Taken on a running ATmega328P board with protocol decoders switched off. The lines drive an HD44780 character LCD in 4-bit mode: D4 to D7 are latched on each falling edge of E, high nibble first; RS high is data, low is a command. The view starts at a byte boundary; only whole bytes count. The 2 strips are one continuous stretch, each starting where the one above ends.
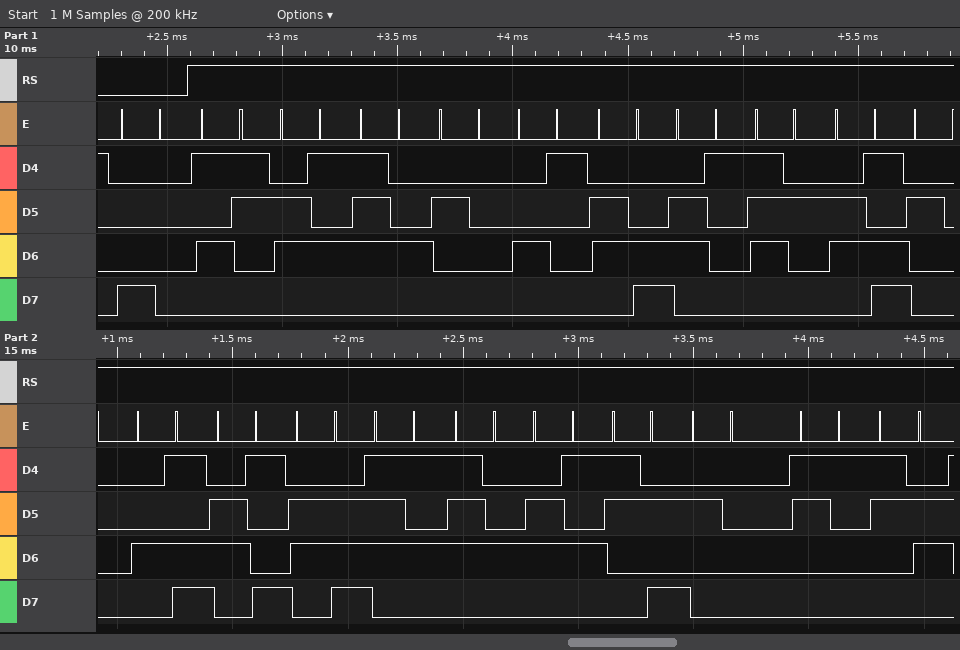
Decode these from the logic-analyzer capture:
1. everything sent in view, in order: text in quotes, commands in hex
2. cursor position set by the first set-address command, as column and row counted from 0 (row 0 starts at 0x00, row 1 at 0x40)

0x80 "Set Alarm Minute: 16"
column 0, row 0
